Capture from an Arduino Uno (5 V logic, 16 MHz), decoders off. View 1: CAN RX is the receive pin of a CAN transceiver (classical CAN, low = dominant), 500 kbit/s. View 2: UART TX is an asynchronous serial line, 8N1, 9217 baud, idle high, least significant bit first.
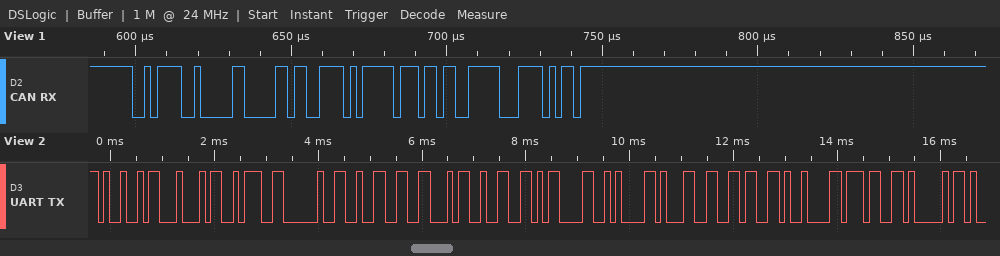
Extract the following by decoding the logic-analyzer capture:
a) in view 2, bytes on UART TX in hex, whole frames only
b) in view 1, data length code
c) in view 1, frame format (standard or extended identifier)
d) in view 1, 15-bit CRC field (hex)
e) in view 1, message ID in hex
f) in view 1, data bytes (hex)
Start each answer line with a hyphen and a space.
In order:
- 49 44 3A 20 32 46 32 0D 0A 31 36 09 37 41
- 4
- standard
- 0x7CF5
- 0x2F2
- 16 7A FF 6C
